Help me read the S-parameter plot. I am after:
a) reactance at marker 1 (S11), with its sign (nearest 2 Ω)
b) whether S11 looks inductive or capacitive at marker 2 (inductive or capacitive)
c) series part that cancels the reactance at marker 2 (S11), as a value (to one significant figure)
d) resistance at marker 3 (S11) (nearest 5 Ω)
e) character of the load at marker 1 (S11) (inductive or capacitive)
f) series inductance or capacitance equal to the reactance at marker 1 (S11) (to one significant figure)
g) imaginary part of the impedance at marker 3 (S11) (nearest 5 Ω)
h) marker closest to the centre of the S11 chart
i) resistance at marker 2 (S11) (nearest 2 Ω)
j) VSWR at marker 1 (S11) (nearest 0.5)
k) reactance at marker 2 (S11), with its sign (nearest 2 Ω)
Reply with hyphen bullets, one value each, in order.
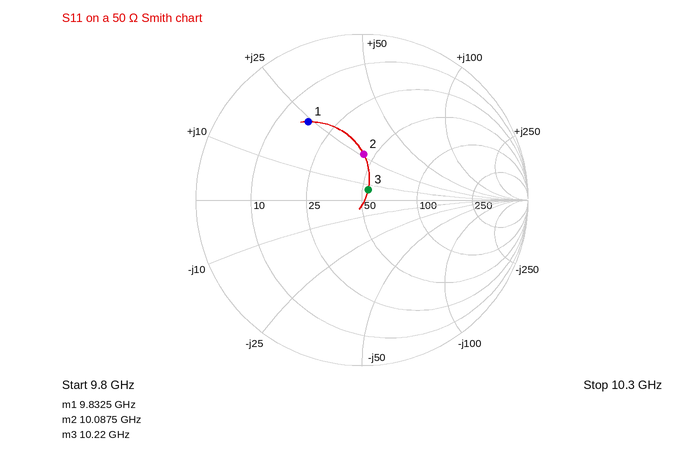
- +24 Ω
- inductive
- 600 fF
- 55 Ω
- inductive
- 400 pH
- +5 Ω
- marker 3
- 44 Ω
- 3.5
- +26 Ω
